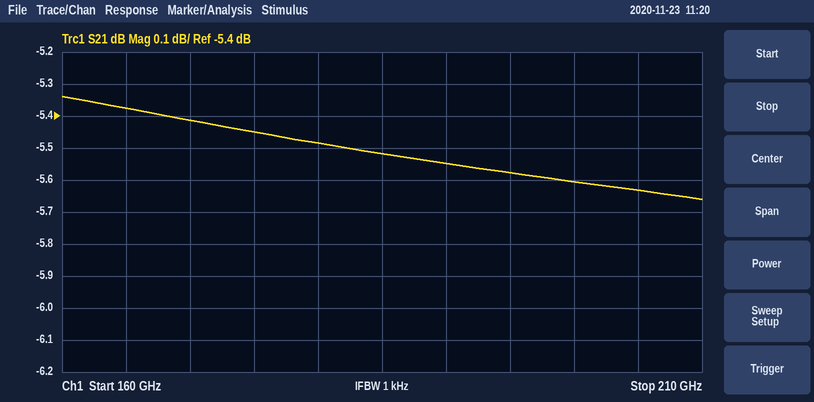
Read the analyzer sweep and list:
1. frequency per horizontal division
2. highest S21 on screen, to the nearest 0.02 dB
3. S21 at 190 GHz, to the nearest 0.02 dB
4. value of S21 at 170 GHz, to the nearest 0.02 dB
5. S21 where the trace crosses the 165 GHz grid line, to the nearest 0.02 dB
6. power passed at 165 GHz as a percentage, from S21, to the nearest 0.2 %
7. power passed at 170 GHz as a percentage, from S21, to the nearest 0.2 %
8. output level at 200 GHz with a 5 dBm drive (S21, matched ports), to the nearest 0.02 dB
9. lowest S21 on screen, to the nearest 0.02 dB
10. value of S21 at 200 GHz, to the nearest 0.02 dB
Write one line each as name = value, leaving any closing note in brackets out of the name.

frequency per horizontal division = 5 GHz
highest S21 on screen, to the nearest 0.02 dB = -5.34 dB
S21 at 190 GHz, to the nearest 0.02 dB = -5.54 dB
value of S21 at 170 GHz, to the nearest 0.02 dB = -5.42 dB
S21 where the trace crosses the 165 GHz grid line, to the nearest 0.02 dB = -5.38 dB
power passed at 165 GHz as a percentage, from S21, to the nearest 0.2 % = 29.0 %
power passed at 170 GHz as a percentage, from S21, to the nearest 0.2 % = 28.8 %
output level at 200 GHz with a 5 dBm drive (S21, matched ports), to the nearest 0.02 dB = -0.60 dBm
lowest S21 on screen, to the nearest 0.02 dB = -5.66 dB
value of S21 at 200 GHz, to the nearest 0.02 dB = -5.60 dB
